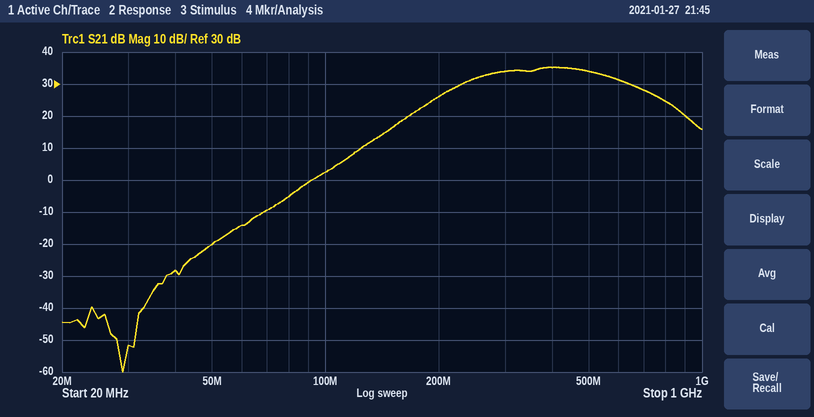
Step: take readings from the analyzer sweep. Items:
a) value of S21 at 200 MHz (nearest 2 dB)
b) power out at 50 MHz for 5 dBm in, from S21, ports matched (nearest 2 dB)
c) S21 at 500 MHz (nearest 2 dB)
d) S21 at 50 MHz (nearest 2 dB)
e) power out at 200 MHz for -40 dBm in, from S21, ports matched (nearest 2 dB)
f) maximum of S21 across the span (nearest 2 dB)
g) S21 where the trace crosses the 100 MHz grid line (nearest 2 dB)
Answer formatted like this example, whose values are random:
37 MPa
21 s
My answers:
26 dB
-16 dBm
34 dB
-20 dB
-14 dBm
36 dB
2 dB
